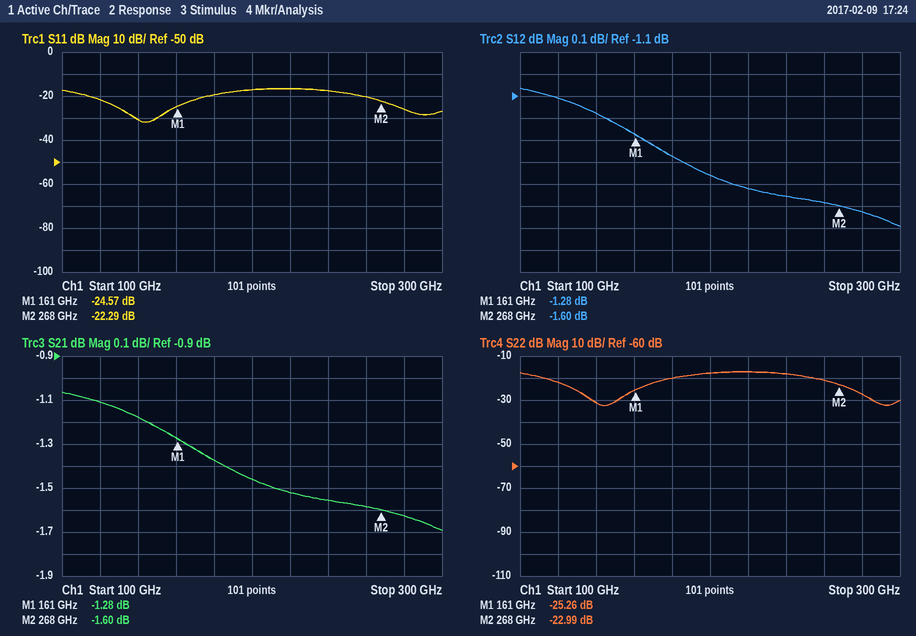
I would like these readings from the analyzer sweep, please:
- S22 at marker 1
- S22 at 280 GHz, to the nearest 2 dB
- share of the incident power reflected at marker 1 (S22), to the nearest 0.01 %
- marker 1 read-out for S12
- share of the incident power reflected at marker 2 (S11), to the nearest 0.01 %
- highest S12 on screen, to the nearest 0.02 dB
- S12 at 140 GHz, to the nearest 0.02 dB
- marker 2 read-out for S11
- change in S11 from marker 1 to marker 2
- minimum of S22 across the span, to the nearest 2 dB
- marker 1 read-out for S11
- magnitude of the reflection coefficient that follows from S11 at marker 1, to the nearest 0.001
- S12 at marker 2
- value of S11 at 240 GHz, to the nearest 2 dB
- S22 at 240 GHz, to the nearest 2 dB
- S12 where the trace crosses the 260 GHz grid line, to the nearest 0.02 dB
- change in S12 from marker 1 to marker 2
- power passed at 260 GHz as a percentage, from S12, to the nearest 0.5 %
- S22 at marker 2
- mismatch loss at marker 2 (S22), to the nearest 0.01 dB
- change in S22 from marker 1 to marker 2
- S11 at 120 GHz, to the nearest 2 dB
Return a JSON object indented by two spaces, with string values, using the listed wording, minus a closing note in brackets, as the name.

{
  "S22 at marker 1": "-25.26 dB",
  "S22 at 280 GHz, to the nearest 2 dB": "-28 dB",
  "share of the incident power reflected at marker 1 (S22), to the nearest 0.01 %": "0.30 %",
  "marker 1 read-out for S12": "-1.28 dB",
  "share of the incident power reflected at marker 2 (S11), to the nearest 0.01 %": "0.59 %",
  "highest S12 on screen, to the nearest 0.02 dB": "-1.06 dB",
  "S12 at 140 GHz, to the nearest 0.02 dB": "-1.18 dB",
  "marker 2 read-out for S11": "-22.29 dB",
  "change in S11 from marker 1 to marker 2": "2.28 dB",
  "minimum of S22 across the span, to the nearest 2 dB": "-32 dB",
  "marker 1 read-out for S11": "-24.57 dB",
  "magnitude of the reflection coefficient that follows from S11 at marker 1, to the nearest 0.001": "0.059",
  "S12 at marker 2": "-1.60 dB",
  "value of S11 at 240 GHz, to the nearest 2 dB": "-18 dB",
  "S22 at 240 GHz, to the nearest 2 dB": "-18 dB",
  "S12 where the trace crosses the 260 GHz grid line, to the nearest 0.02 dB": "-1.58 dB",
  "change in S12 from marker 1 to marker 2": "-0.32 dB",
  "power passed at 260 GHz as a percentage, from S12, to the nearest 0.5 %": "69.5 %",
  "S22 at marker 2": "-22.99 dB",
  "mismatch loss at marker 2 (S22), to the nearest 0.01 dB": "0.02 dB",
  "change in S22 from marker 1 to marker 2": "2.27 dB",
  "S11 at 120 GHz, to the nearest 2 dB": "-22 dB"
}
